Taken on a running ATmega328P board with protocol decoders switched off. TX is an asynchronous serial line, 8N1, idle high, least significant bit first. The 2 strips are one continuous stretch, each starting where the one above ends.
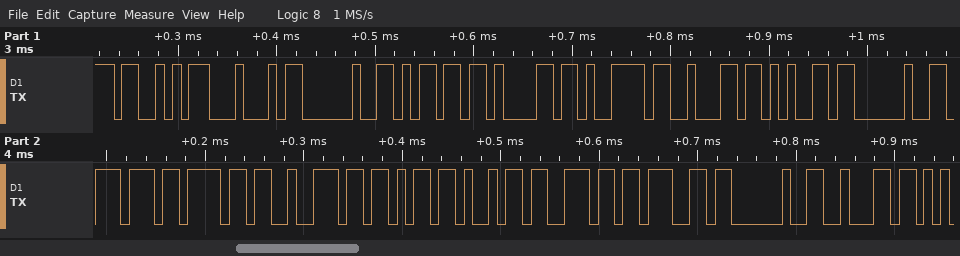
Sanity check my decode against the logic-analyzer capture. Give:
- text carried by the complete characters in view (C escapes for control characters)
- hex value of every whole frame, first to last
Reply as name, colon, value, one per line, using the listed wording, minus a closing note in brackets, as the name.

text carried by the complete characters in view: "SD maybe working b"
hex value of every whole frame, first to last: 0x53 0x44 0x20 0x6D 0x61 0x79 0x62 0x65 0x20 0x77 0x6F 0x72 0x6B 0x69 0x6E 0x67 0x20 0x62
